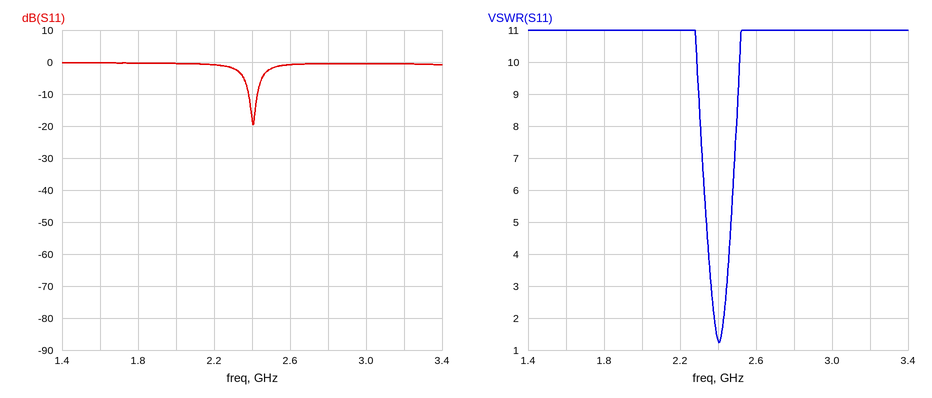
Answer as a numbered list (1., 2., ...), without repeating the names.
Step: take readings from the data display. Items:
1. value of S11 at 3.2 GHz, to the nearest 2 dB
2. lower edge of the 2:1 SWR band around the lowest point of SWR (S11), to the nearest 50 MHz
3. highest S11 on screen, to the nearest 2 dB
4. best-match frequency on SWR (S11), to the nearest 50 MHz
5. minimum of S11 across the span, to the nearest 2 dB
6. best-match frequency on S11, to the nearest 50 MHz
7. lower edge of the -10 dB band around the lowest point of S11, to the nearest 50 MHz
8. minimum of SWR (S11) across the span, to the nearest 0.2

1. 0 dB
2. 2.40 GHz
3. 0 dB
4. 2.40 GHz
5. -20 dB
6. 2.40 GHz
7. 2.40 GHz
8. 1.2
